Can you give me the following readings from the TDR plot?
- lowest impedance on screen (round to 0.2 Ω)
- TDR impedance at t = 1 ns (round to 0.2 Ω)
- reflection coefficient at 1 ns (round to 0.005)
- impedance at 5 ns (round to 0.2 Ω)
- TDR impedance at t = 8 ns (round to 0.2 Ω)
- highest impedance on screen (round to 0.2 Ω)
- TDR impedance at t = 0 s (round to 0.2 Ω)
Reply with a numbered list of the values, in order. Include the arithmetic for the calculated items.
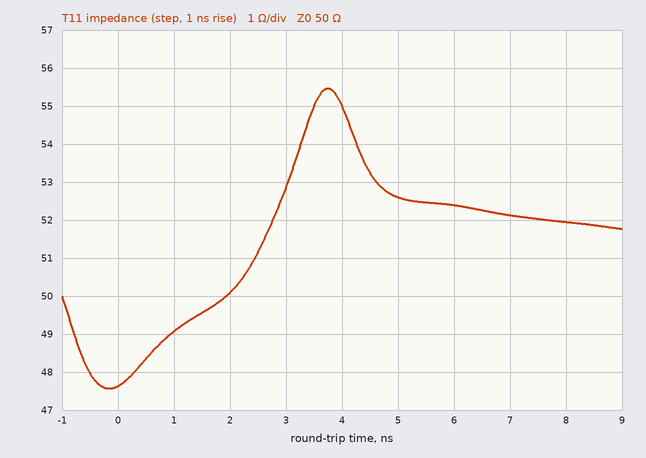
1. 47.6 Ω
2. 49.0 Ω
3. (49 − 50)/(49 + 50) ≈ -0.010
4. 52.6 Ω
5. 52.0 Ω
6. 55.4 Ω
7. 47.6 Ω
